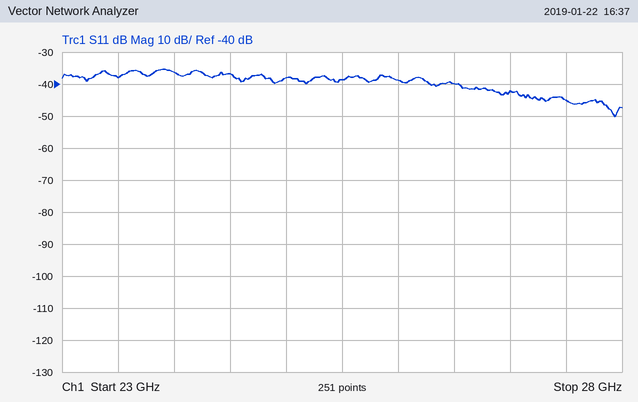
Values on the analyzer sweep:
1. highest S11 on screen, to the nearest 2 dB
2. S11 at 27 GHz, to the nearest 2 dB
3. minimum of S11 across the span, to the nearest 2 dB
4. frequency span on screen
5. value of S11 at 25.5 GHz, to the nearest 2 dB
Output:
-36 dB
-42 dB
-50 dB
5 GHz
-38 dB
